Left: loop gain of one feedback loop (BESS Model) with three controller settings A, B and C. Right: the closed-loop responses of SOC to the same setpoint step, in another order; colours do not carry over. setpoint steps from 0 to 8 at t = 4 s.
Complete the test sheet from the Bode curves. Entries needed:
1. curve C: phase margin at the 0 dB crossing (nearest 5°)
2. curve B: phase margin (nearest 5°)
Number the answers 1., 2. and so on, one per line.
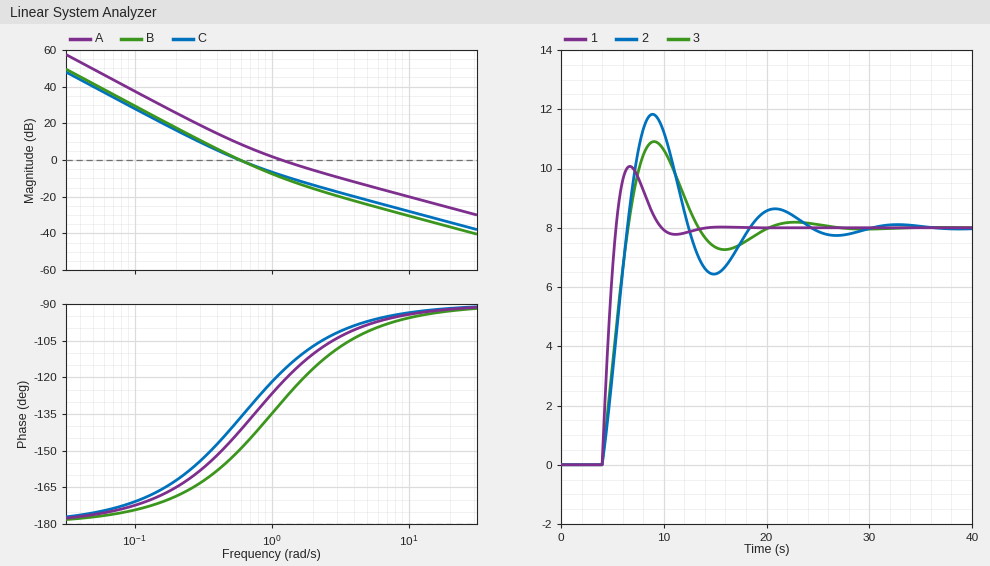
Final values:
1. 45°
2. 30°
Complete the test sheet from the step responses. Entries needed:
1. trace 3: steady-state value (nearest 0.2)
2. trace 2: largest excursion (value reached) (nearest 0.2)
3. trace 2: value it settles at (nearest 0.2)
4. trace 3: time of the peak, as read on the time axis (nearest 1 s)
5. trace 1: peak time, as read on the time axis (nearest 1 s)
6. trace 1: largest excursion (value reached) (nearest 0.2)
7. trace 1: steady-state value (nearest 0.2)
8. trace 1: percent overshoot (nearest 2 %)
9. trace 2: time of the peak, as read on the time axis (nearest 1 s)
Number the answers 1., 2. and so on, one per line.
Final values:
1. 8.0
2. 11.8
3. 8.0
4. 9 s
5. 7 s
6. 10.0
7. 8.0
8. 26 %
9. 9 s
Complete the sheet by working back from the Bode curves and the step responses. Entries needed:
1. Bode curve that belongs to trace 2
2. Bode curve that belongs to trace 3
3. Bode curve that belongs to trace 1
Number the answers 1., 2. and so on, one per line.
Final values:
1. B
2. C
3. A
